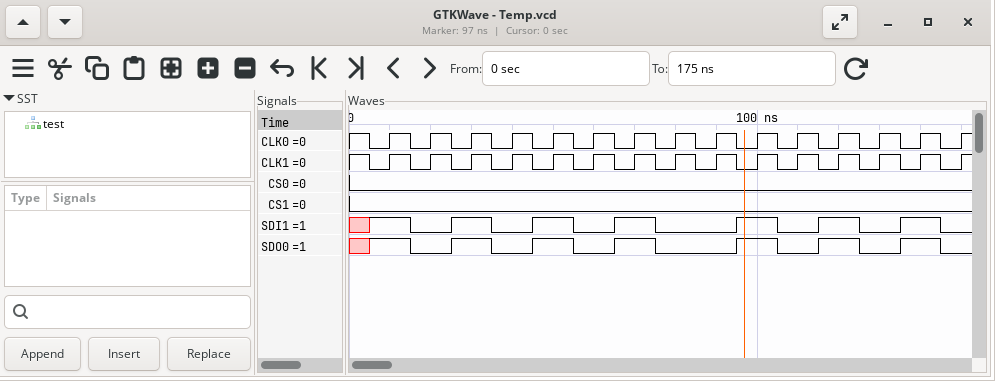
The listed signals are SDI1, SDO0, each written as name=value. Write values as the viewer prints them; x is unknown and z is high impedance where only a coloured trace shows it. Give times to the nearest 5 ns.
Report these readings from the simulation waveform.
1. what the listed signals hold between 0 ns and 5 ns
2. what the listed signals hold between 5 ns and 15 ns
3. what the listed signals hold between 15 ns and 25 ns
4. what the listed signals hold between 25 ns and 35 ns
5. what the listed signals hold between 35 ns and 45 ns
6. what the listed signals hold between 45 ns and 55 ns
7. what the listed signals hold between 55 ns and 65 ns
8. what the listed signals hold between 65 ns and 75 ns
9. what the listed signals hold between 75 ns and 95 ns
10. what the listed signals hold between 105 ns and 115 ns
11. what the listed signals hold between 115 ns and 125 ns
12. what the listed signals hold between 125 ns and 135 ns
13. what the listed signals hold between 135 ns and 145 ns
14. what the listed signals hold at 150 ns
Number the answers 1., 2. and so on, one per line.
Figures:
1. SDI1=x, SDO0=x
2. SDI1=1, SDO0=1
3. SDI1=0, SDO0=0
4. SDI1=1, SDO0=1
5. SDI1=0, SDO0=0
6. SDI1=1, SDO0=1
7. SDI1=0, SDO0=0
8. SDI1=1, SDO0=1
9. SDI1=0, SDO0=0
10. SDI1=0, SDO0=0
11. SDI1=1, SDO0=1
12. SDI1=0, SDO0=0
13. SDI1=1, SDO0=1
14. SDI1=0, SDO0=0
